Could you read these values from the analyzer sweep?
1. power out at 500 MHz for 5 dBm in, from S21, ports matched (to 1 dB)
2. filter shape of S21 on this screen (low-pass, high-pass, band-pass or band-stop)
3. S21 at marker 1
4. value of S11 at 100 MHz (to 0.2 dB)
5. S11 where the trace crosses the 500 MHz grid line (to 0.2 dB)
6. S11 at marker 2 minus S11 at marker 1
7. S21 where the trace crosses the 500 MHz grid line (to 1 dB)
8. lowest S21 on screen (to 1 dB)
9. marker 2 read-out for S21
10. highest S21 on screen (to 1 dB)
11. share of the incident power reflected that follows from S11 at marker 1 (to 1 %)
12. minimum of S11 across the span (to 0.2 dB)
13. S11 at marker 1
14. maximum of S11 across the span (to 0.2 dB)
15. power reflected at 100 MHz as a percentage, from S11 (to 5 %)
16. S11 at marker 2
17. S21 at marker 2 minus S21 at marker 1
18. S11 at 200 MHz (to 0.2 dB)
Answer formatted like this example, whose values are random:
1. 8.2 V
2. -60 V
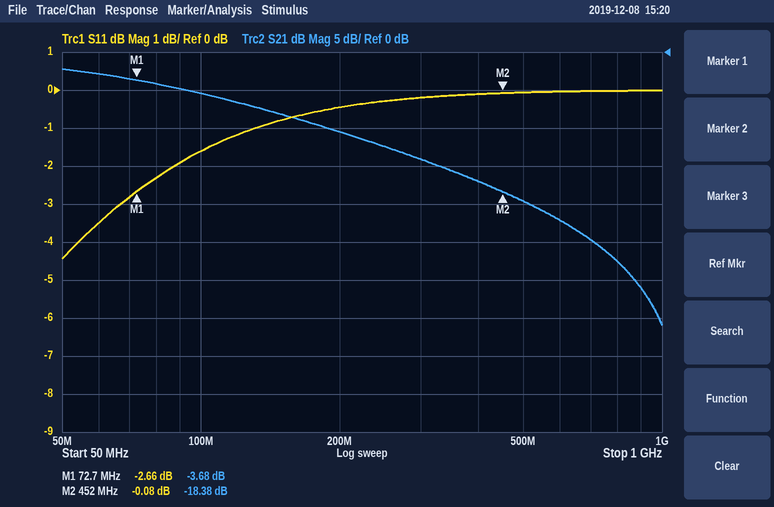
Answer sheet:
1. -15 dBm
2. low-pass
3. -3.68 dB
4. -1.6 dB
5. 0.0 dB
6. 2.58 dB
7. -20 dB
8. -36 dB
9. -18.38 dB
10. -2 dB
11. 54 %
12. -4.4 dB
13. -2.66 dB
14. 0.0 dB
15. 70 %
16. -0.08 dB
17. -14.70 dB
18. -0.4 dB
